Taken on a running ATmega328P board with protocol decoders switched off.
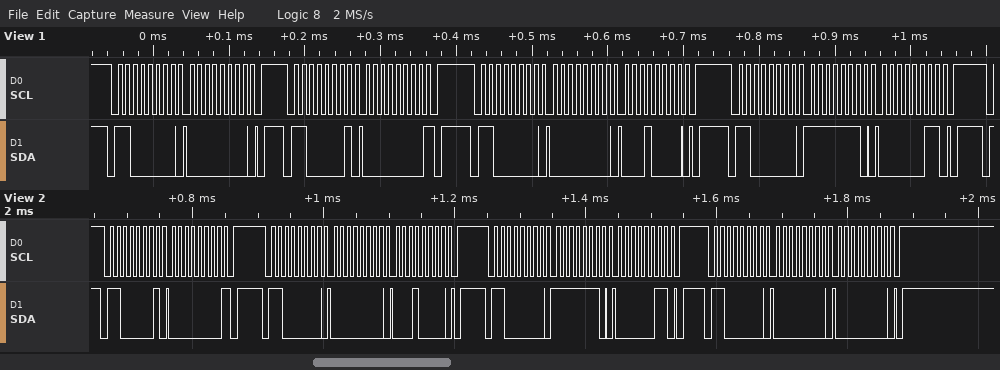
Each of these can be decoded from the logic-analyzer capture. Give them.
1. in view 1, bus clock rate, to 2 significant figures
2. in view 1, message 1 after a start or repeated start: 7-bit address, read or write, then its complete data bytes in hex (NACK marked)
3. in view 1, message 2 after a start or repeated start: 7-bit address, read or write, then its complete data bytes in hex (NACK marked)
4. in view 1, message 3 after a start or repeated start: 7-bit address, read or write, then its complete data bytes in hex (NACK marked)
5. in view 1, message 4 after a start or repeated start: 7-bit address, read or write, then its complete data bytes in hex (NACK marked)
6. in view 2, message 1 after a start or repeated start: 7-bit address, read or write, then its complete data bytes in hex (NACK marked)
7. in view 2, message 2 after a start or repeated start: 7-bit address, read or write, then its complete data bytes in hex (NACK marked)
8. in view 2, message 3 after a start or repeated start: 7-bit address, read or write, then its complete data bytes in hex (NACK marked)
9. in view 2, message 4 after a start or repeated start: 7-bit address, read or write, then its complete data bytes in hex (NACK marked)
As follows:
100 kHz
0x60 write: 00
0x60 read: 00 NACK
0x60 write: 00 10
0x60 write: FE 03
0x60 read: 00 NACK
0x60 write: 00 10
0x60 write: FE 03
0x60 write: 00 00
